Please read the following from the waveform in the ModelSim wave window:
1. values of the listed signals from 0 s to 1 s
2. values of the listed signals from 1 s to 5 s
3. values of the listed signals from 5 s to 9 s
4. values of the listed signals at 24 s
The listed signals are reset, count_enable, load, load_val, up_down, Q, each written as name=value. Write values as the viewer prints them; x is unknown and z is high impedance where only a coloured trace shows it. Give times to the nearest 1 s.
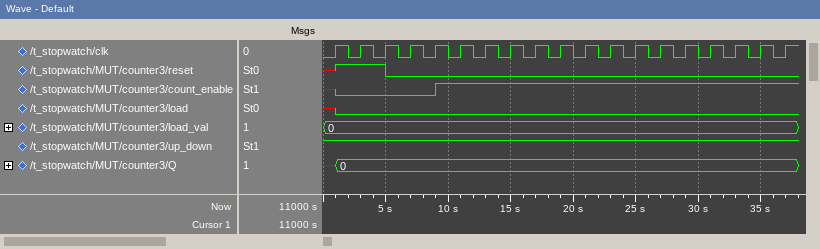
reset=x, count_enable=x, load=x, load_val=0, up_down=1, Q=x
reset=1, count_enable=0, load=0, load_val=0, up_down=1, Q=0
reset=0, count_enable=0, load=0, load_val=0, up_down=1, Q=0
reset=0, count_enable=1, load=0, load_val=0, up_down=1, Q=0
